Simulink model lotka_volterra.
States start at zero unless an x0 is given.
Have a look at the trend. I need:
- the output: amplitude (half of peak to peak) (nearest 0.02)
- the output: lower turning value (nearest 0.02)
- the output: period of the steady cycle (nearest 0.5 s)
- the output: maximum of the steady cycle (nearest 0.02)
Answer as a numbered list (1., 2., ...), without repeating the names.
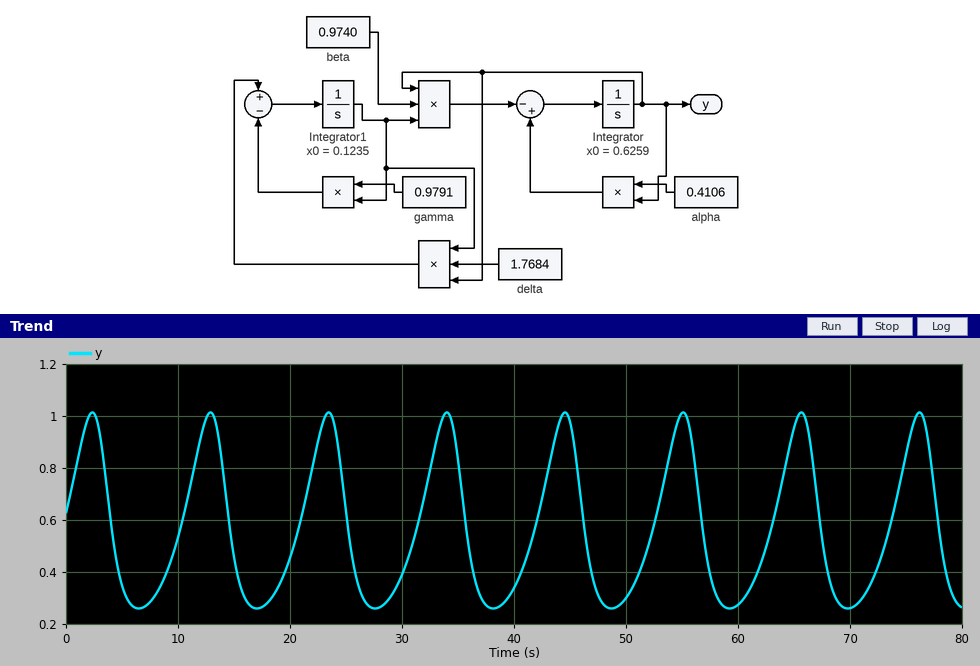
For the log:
1. 0.38
2. 0.26
3. 10.5 s
4. 1.02
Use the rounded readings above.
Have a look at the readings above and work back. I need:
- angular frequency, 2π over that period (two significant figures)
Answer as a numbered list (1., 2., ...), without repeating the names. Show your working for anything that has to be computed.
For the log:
1. 2π / 10.5 = 0.60 rad/s
